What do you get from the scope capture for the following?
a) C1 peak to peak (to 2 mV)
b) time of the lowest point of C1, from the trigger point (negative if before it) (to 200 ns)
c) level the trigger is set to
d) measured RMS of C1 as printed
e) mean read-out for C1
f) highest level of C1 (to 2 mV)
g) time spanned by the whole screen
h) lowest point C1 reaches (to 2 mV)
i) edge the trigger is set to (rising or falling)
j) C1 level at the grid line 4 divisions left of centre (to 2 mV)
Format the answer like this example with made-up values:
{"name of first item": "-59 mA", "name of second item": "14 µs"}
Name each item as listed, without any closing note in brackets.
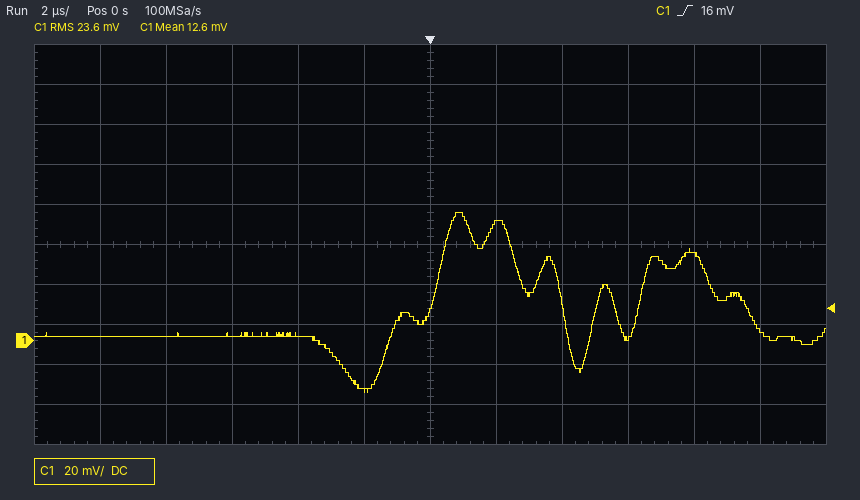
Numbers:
{"C1 peak to peak": "90 mV", "time of the lowest point of C1, from the trigger point (negative if before it)": "-2.0 µs", "level the trigger is set to": "16 mV", "measured RMS of C1 as printed": "23.6 mV", "mean read-out for C1": "12.6 mV", "highest level of C1": "64 mV", "time spanned by the whole screen": "24 µs", "lowest point C1 reaches": "-26 mV", "edge the trigger is set to": "rising", "C1 level at the grid line 4 divisions left of centre": "2 mV"}
